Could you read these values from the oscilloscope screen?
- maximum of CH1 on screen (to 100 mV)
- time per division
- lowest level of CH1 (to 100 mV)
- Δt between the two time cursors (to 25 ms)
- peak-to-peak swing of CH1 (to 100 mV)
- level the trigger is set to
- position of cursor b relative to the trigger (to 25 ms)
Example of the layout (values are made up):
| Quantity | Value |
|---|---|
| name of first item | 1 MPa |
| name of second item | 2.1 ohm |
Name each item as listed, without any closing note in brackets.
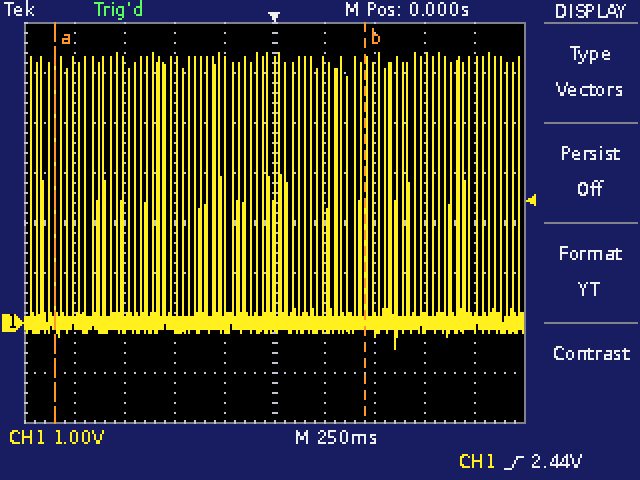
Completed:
| Quantity | Value |
|---|---|
| maximum of CH1 on screen | 5.4 V |
| time per division | 250 ms |
| lowest level of CH1 | -500 mV |
| Δt between the two time cursors | 1.550 s |
| peak-to-peak swing of CH1 | 5.9 V |
| level the trigger is set to | 2.44 V |
| position of cursor b relative to the trigger | +450 ms |
